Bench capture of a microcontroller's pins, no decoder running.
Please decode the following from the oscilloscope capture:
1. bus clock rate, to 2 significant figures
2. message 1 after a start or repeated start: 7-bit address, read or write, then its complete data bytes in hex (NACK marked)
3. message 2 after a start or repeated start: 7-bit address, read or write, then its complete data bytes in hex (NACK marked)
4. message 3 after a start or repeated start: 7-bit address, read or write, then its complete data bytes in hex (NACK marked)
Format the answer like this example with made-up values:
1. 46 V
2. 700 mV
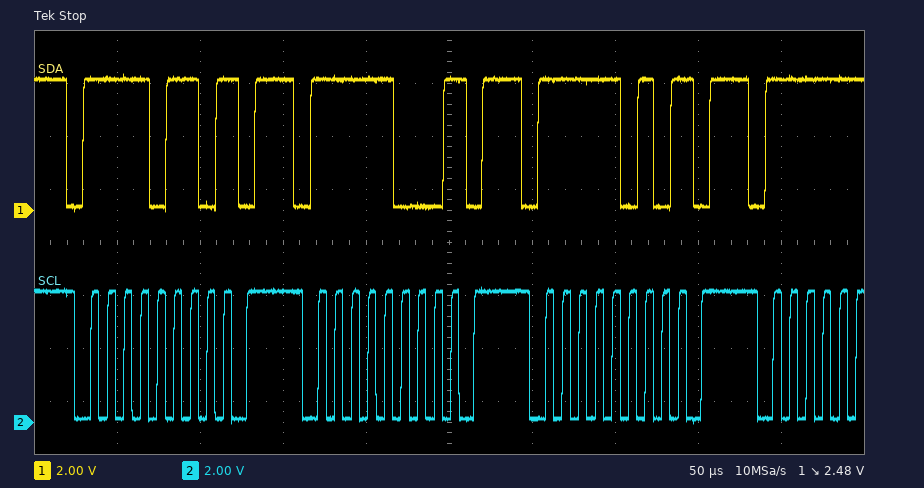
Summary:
1. 100 kHz
2. 0x7B write NACK
3. 0x7C write NACK
4. 0x7D write NACK
